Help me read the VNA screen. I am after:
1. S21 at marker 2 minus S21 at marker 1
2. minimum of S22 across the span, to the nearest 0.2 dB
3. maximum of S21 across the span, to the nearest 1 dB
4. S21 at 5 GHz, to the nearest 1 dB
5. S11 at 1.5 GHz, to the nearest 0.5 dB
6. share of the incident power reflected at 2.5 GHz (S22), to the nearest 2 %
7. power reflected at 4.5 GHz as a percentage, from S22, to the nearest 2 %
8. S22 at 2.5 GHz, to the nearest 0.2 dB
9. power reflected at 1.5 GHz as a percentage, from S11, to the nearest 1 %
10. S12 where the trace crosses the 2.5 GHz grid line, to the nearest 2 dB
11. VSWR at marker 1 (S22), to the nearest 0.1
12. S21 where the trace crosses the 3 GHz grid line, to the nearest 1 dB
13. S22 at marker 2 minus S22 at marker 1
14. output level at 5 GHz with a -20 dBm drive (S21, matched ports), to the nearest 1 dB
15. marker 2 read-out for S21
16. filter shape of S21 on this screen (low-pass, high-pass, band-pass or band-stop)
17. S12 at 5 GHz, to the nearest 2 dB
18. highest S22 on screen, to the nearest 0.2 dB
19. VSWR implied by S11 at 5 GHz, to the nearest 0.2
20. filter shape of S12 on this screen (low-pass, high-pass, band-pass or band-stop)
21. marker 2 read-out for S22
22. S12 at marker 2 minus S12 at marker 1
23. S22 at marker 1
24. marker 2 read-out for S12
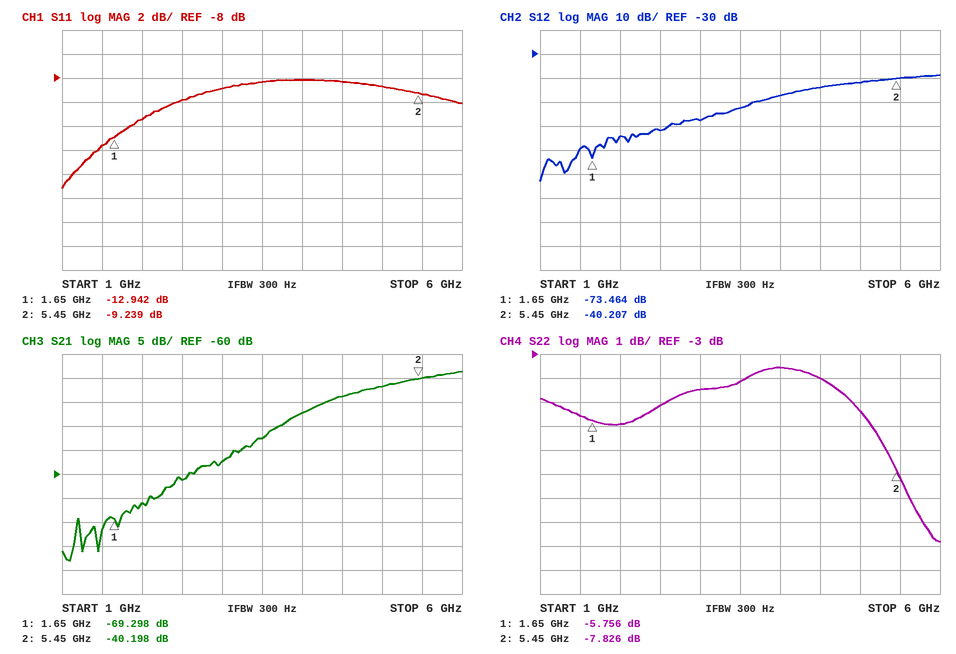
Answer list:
29.100 dB
-10.8 dB
-39 dB
-42 dB
-13.5 dB
30 %
40 %
-5.2 dB
4 %
-62 dB
3.1
-57 dB
-2.070 dB
-62 dBm
-40.198 dB
high-pass
-42 dB
-3.6 dB
2.2
high-pass
-7.826 dB
33.257 dB
-5.756 dB
-40.207 dB
